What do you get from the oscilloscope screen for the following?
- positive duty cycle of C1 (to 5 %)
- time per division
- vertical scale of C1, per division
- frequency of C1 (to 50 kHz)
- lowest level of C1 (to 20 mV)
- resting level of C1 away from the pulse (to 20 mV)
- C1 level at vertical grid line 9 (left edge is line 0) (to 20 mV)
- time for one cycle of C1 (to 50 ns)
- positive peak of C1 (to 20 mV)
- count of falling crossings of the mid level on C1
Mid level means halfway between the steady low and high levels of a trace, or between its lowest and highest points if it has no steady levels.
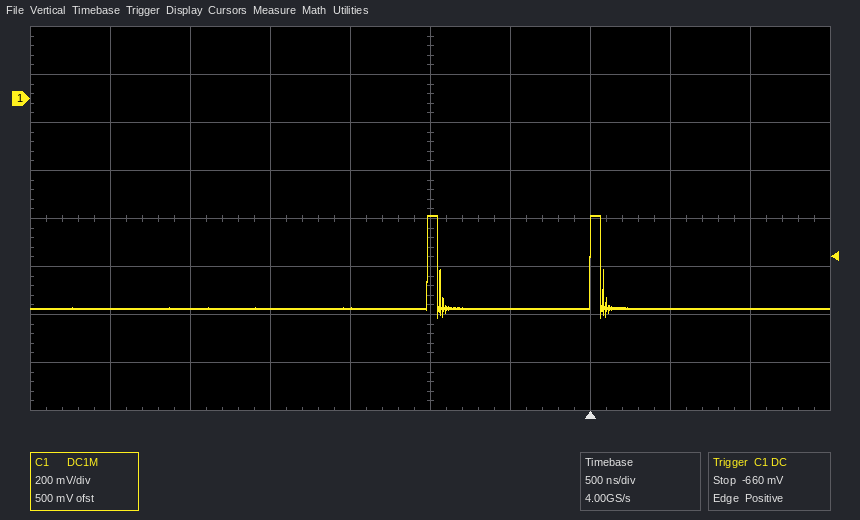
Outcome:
5 %
500 ns
200 mV
1.00 MHz
-920 mV
-880 mV
-880 mV
1.00 µs
-480 mV
2
